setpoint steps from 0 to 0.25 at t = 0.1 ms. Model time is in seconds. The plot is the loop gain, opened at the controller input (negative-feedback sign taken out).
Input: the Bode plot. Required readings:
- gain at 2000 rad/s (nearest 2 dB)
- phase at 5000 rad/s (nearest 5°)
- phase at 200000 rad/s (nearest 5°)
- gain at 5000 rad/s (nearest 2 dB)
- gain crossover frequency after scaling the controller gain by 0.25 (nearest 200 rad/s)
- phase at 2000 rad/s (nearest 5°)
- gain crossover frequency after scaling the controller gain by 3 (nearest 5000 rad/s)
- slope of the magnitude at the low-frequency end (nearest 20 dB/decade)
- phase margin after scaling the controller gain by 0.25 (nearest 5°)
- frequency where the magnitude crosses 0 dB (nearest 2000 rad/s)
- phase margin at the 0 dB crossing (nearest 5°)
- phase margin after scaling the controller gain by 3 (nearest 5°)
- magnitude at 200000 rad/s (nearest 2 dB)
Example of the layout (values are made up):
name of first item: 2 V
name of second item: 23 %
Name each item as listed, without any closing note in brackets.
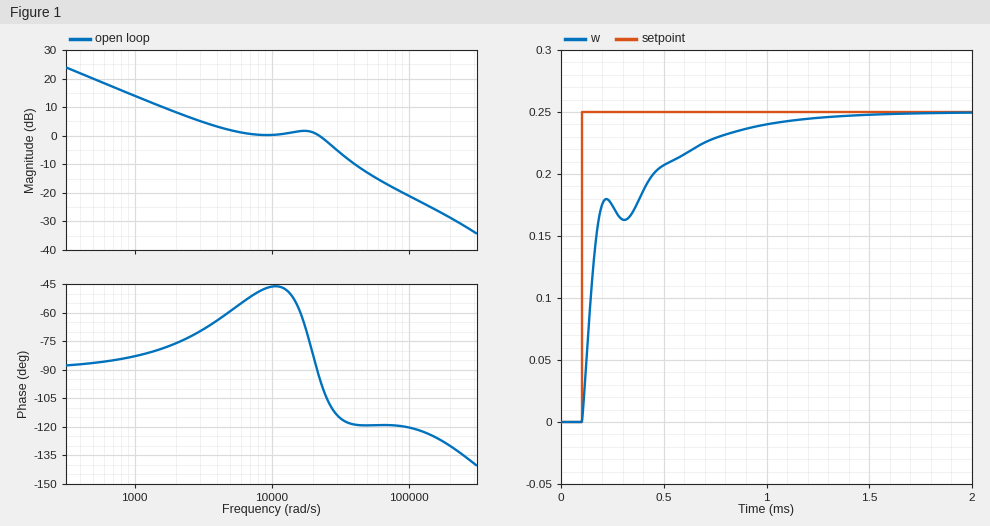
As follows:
gain at 2000 rad/s: 8 dB
phase at 5000 rad/s: -60°
phase at 200000 rad/s: -130°
gain at 5000 rad/s: 2 dB
gain crossover frequency after scaling the controller gain by 0.25: 1200 rad/s
phase at 2000 rad/s: -75°
gain crossover frequency after scaling the controller gain by 3: 40000 rad/s
slope of the magnitude at the low-frequency end: -20 dB/decade
phase margin after scaling the controller gain by 0.25: 100°
frequency where the magnitude crosses 0 dB: 22000 rad/s
phase margin at the 0 dB crossing: 85°
phase margin after scaling the controller gain by 3: 60°
magnitude at 200000 rad/s: -28 dB
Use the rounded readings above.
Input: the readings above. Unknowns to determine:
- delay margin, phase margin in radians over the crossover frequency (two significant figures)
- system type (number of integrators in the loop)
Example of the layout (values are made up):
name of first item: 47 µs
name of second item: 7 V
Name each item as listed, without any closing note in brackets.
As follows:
delay margin, phase margin in radians over the crossover frequency: 0.000067 s
system type: 1
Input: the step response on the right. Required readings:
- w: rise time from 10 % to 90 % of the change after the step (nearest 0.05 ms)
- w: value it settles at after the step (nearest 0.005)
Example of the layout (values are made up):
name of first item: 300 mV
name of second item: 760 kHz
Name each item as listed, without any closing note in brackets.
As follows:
w: rise time from 10 % to 90 % of the change after the step: 0.60 ms
w: value it settles at after the step: 0.250
